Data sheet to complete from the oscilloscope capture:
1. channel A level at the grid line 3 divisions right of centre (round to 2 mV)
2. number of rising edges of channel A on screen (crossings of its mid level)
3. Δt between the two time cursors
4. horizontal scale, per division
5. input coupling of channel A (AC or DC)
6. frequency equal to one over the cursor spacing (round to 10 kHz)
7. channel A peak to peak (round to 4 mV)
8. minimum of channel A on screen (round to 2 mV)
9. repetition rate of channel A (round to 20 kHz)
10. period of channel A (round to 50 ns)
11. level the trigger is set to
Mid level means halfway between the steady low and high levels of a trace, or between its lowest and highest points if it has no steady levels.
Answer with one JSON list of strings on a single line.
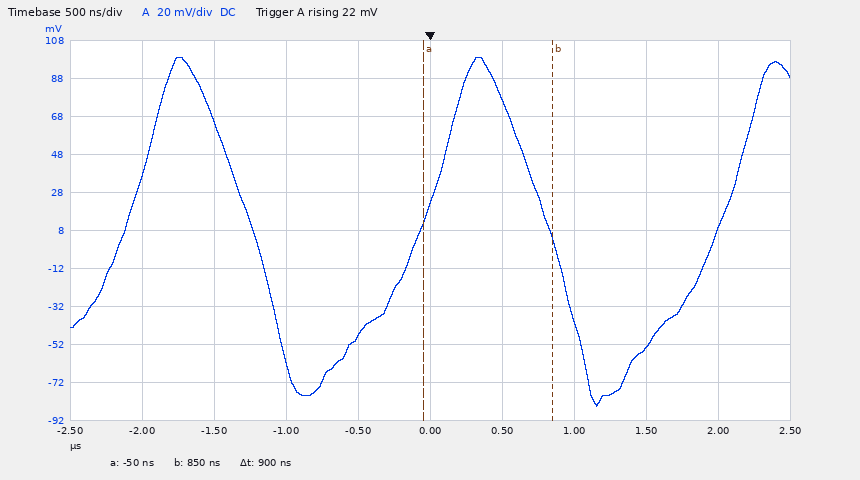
["-54 mV", "3", "900 ns", "500 ns", "DC", "1.11 MHz", "184 mV", "-84 mV", "480 kHz", "2.05 µs", "22 mV"]
